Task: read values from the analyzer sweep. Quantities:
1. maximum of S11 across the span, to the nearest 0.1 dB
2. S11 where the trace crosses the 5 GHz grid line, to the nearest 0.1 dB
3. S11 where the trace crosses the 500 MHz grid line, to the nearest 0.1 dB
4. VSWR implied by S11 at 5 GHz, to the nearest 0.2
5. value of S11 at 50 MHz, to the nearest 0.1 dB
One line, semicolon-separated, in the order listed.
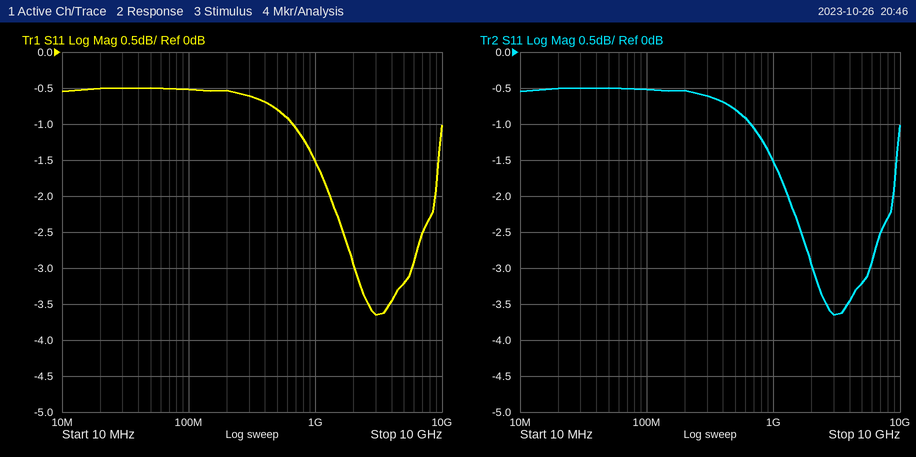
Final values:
-0.5 dB; -3.2 dB; -0.8 dB; 5.4; -0.5 dB
